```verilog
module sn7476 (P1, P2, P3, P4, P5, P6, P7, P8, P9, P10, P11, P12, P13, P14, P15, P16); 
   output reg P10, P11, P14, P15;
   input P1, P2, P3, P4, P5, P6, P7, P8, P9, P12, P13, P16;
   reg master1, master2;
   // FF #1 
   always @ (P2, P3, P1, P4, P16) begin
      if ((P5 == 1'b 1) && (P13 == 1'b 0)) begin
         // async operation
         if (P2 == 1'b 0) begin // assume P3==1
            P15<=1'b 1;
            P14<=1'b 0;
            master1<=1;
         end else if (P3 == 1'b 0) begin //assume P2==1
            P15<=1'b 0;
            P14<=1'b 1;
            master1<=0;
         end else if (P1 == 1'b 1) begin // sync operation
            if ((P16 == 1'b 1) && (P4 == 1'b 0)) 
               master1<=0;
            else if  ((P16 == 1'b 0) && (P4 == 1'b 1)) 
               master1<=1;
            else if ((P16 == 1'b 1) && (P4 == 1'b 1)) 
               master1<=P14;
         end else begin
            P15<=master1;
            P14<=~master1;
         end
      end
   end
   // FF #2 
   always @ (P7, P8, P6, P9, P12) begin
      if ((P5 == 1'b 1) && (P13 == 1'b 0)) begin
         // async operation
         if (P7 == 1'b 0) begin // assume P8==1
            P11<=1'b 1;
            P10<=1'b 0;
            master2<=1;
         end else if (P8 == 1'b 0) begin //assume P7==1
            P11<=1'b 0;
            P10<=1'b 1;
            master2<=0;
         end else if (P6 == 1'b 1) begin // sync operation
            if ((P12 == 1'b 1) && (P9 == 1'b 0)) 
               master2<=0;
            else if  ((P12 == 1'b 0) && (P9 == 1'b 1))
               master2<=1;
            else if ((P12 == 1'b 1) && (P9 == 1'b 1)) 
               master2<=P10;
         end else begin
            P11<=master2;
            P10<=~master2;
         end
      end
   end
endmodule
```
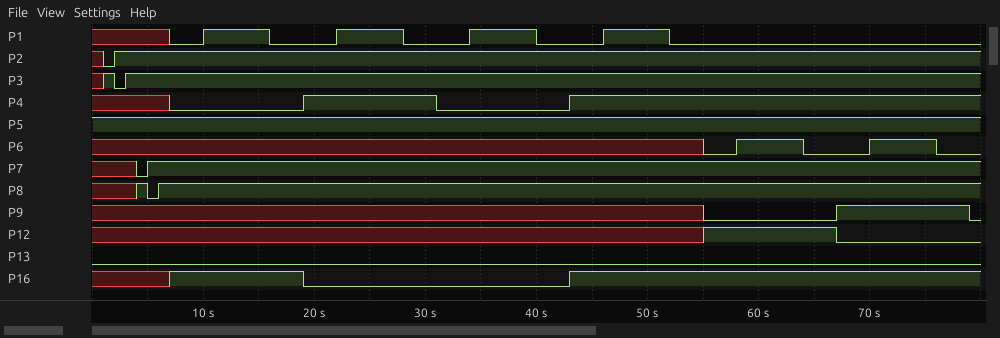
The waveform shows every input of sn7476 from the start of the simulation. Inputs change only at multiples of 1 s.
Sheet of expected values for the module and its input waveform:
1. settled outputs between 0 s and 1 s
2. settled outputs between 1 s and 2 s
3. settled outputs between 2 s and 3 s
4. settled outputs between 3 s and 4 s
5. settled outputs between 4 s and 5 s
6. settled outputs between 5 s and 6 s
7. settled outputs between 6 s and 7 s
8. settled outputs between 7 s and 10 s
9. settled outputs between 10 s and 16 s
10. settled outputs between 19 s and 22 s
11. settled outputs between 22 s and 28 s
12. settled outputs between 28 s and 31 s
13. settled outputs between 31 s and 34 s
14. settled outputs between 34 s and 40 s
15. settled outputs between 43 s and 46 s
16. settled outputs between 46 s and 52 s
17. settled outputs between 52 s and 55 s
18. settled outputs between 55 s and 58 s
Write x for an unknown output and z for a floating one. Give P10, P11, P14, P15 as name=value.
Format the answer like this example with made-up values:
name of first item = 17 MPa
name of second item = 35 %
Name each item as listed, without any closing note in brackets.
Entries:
settled outputs between 0 s and 1 s = P10=x, P11=x, P14=x, P15=x
settled outputs between 1 s and 2 s = P10=x, P11=x, P14=0, P15=1
settled outputs between 2 s and 3 s = P10=x, P11=x, P14=1, P15=0
settled outputs between 3 s and 4 s = P10=x, P11=x, P14=1, P15=0
settled outputs between 4 s and 5 s = P10=0, P11=1, P14=1, P15=0
settled outputs between 5 s and 6 s = P10=1, P11=0, P14=1, P15=0
settled outputs between 6 s and 7 s = P10=1, P11=0, P14=1, P15=0
settled outputs between 7 s and 10 s = P10=1, P11=0, P14=1, P15=0
settled outputs between 10 s and 16 s = P10=1, P11=0, P14=1, P15=0
settled outputs between 19 s and 22 s = P10=1, P11=0, P14=1, P15=0
settled outputs between 22 s and 28 s = P10=1, P11=0, P14=1, P15=0
settled outputs between 28 s and 31 s = P10=1, P11=0, P14=0, P15=1
settled outputs between 31 s and 34 s = P10=1, P11=0, P14=0, P15=1
settled outputs between 34 s and 40 s = P10=1, P11=0, P14=0, P15=1
settled outputs between 43 s and 46 s = P10=1, P11=0, P14=0, P15=1
settled outputs between 46 s and 52 s = P10=1, P11=0, P14=0, P15=1
settled outputs between 52 s and 55 s = P10=1, P11=0, P14=1, P15=0
settled outputs between 55 s and 58 s = P10=1, P11=0, P14=1, P15=0
